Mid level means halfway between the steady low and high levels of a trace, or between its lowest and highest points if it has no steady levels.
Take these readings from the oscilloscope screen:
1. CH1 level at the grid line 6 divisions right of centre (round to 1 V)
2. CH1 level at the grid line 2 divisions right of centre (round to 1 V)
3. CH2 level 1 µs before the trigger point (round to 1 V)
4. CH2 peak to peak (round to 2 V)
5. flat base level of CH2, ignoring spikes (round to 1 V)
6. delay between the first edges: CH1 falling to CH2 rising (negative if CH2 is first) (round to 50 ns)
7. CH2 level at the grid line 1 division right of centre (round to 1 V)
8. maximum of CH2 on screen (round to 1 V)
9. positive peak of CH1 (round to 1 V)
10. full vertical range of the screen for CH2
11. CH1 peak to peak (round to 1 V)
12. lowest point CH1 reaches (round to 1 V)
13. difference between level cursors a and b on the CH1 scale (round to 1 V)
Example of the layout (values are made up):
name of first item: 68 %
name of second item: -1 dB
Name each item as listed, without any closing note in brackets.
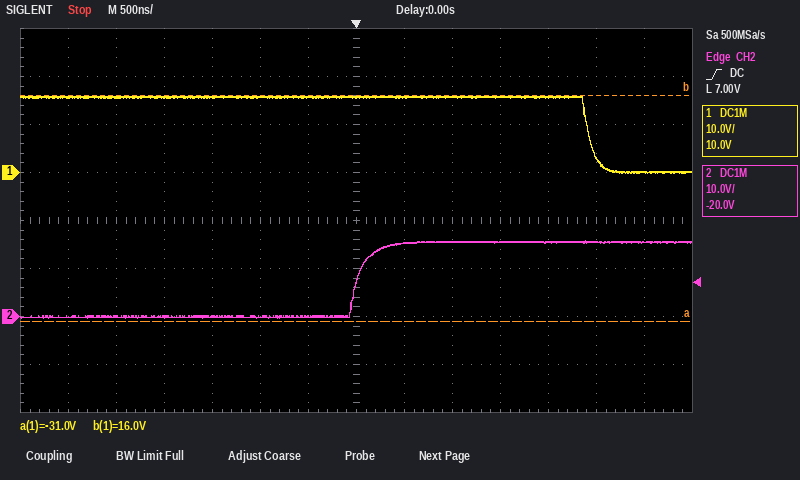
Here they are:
CH1 level at the grid line 6 divisions right of centre: 0 V
CH1 level at the grid line 2 divisions right of centre: 16 V
CH2 level 1 µs before the trigger point: 0 V
CH2 peak to peak: 16 V
flat base level of CH2, ignoring spikes: 0 V
delay between the first edges: CH1 falling to CH2 rising (negative if CH2 is first): -2.40 µs
CH2 level at the grid line 1 division right of centre: 15 V
maximum of CH2 on screen: 16 V
positive peak of CH1: 16 V
full vertical range of the screen for CH2: 80 V
CH1 peak to peak: 16 V
lowest point CH1 reaches: 0 V
difference between level cursors a and b on the CH1 scale: 47 V
